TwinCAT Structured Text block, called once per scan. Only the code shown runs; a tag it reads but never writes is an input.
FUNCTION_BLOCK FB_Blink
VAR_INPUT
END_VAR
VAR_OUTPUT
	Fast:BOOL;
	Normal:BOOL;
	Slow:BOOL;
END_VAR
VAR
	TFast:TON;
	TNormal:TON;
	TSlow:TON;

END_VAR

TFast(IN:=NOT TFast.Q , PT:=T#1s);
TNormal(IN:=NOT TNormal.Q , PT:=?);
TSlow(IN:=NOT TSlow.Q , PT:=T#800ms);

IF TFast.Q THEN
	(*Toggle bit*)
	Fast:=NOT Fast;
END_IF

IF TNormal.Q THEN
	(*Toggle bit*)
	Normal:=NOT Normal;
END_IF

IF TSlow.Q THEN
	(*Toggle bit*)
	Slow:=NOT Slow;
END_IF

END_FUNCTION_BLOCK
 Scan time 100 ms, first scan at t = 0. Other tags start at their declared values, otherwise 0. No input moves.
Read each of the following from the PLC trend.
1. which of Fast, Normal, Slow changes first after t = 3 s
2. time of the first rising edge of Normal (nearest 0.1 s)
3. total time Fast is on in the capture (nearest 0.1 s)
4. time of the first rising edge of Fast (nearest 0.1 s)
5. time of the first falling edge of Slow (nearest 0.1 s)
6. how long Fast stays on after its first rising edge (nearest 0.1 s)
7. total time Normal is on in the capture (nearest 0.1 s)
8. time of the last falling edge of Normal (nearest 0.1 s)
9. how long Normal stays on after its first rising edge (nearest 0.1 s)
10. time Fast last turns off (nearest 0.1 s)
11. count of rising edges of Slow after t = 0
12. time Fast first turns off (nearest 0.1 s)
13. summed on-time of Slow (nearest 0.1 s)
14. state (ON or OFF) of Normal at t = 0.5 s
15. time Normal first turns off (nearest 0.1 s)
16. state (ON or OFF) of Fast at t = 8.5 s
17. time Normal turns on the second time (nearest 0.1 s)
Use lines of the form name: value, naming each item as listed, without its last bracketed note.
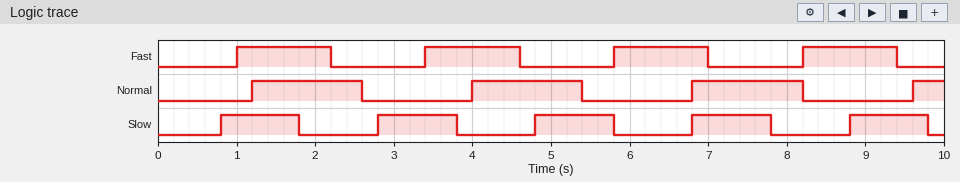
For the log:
which of Fast, Normal, Slow changes first after t = 3 s: Fast
time of the first rising edge of Normal: 1.2 s
total time Fast is on in the capture: 4.8 s
time of the first rising edge of Fast: 1.0 s
time of the first falling edge of Slow: 1.8 s
how long Fast stays on after its first rising edge: 1.2 s
total time Normal is on in the capture: 4.6 s
time of the last falling edge of Normal: 8.2 s
how long Normal stays on after its first rising edge: 1.4 s
time Fast last turns off: 9.4 s
count of rising edges of Slow after t = 0: 5
time Fast first turns off: 2.2 s
summed on-time of Slow: 5.0 s
state (ON or OFF) of Normal at t = 0.5 s: OFF
time Normal first turns off: 2.6 s
state (ON or OFF) of Fast at t = 8.5 s: ON
time Normal turns on the second time: 4.0 s
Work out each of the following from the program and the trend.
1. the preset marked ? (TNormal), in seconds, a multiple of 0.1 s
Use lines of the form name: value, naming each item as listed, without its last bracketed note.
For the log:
the preset marked ? (TNormal), in seconds, a multiple of 0.1 s: 1.2 s
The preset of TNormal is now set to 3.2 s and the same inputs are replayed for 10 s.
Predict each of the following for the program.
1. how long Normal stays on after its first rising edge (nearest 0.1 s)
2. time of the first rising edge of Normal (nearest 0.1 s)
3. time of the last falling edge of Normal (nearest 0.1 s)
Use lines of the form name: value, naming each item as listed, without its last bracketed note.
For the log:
how long Normal stays on after its first rising edge: 3.4 s
time of the first rising edge of Normal: 3.2 s
time of the last falling edge of Normal: 6.6 s
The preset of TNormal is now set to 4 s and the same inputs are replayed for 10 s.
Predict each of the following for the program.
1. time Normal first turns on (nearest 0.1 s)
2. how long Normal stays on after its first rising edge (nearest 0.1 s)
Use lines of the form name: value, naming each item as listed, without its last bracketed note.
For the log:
time Normal first turns on: 4.0 s
how long Normal stays on after its first rising edge: 4.2 s
